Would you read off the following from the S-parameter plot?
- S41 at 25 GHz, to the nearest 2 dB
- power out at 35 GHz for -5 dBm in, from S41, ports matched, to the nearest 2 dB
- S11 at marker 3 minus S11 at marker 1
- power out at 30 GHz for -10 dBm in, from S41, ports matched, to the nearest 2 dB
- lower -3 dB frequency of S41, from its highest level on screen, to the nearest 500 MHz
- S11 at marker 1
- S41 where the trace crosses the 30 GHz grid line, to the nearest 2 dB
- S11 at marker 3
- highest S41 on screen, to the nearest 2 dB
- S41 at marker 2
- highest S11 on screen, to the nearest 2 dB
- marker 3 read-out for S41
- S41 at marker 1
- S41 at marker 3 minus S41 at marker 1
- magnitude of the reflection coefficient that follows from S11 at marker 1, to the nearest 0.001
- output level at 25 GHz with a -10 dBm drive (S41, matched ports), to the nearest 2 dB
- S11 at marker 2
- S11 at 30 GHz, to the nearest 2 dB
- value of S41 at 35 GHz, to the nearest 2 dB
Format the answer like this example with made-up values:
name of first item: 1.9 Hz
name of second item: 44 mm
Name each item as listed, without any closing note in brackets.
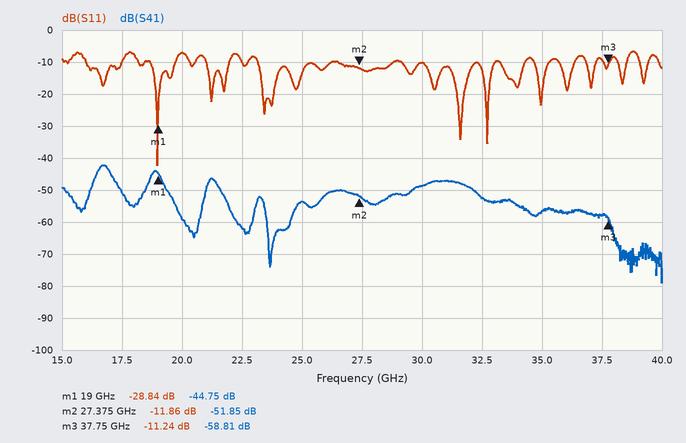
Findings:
S41 at 25 GHz, to the nearest 2 dB: -54 dB
power out at 35 GHz for -5 dBm in, from S41, ports matched, to the nearest 2 dB: -62 dBm
S11 at marker 3 minus S11 at marker 1: 17.60 dB
power out at 30 GHz for -10 dBm in, from S41, ports matched, to the nearest 2 dB: -58 dBm
lower -3 dB frequency of S41, from its highest level on screen, to the nearest 500 MHz: 16.5 GHz
S11 at marker 1: -28.84 dB
S41 where the trace crosses the 30 GHz grid line, to the nearest 2 dB: -48 dB
S11 at marker 3: -11.24 dB
highest S41 on screen, to the nearest 2 dB: -42 dB
S41 at marker 2: -51.85 dB
highest S11 on screen, to the nearest 2 dB: -6 dB
marker 3 read-out for S41: -58.81 dB
S41 at marker 1: -44.75 dB
S41 at marker 3 minus S41 at marker 1: -14.06 dB
magnitude of the reflection coefficient that follows from S11 at marker 1, to the nearest 0.001: 0.036
output level at 25 GHz with a -10 dBm drive (S41, matched ports), to the nearest 2 dB: -64 dBm
S11 at marker 2: -11.86 dB
S11 at 30 GHz, to the nearest 2 dB: -10 dB
value of S41 at 35 GHz, to the nearest 2 dB: -56 dB
